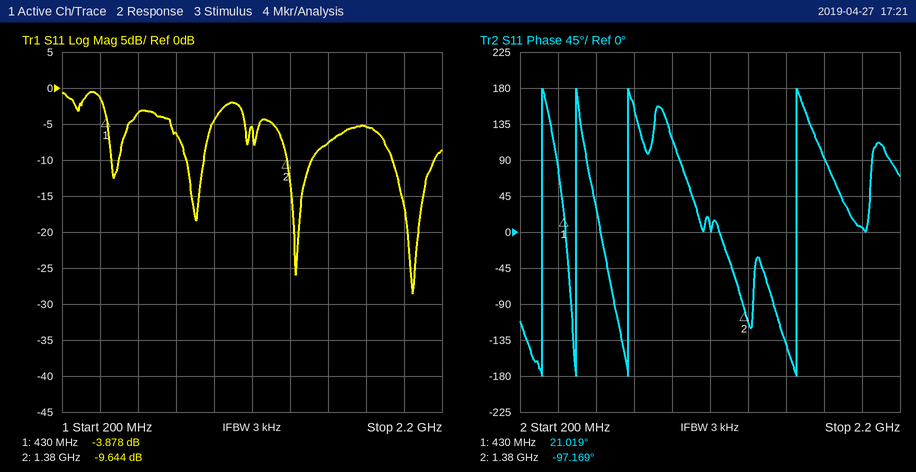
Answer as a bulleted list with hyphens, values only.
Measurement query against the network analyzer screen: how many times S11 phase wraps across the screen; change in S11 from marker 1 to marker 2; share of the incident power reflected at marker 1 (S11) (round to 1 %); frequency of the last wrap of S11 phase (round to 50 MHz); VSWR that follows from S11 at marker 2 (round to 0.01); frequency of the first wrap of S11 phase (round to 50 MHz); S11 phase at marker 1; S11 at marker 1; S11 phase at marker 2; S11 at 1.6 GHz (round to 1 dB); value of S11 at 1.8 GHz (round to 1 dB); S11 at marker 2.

- 4
- -5.766 dB
- 41 %
- 1.65 GHz
- 1.98
- 300 MHz
- 21.019°
- -3.878 dB
- -97.169°
- -8 dB
- -5 dB
- -9.644 dB
